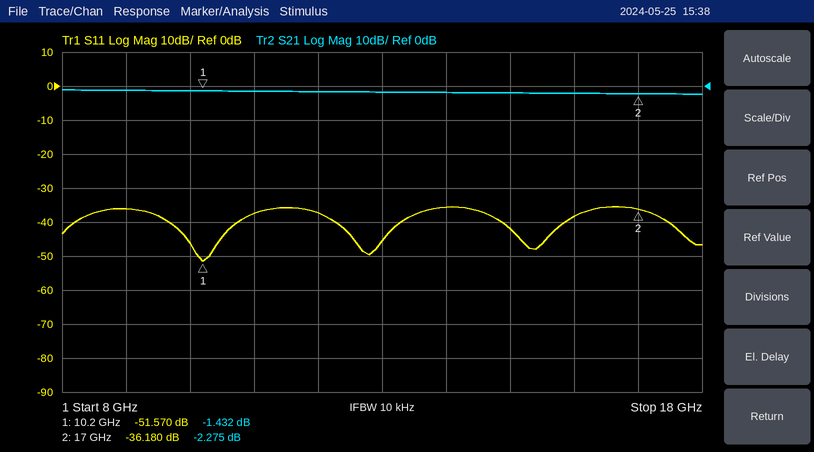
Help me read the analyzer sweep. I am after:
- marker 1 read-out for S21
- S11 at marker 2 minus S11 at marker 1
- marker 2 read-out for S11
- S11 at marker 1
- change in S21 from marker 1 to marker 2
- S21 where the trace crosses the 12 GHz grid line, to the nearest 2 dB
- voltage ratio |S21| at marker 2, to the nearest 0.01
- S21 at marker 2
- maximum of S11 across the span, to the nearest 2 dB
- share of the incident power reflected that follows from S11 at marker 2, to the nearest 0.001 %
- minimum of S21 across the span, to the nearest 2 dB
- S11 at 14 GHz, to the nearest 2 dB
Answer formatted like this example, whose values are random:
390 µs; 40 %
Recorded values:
-1.432 dB; 15.390 dB; -36.180 dB; -51.570 dB; -0.843 dB; -2 dB; 0.77; -2.275 dB; -36 dB; 0.024 %; -2 dB; -36 dB
